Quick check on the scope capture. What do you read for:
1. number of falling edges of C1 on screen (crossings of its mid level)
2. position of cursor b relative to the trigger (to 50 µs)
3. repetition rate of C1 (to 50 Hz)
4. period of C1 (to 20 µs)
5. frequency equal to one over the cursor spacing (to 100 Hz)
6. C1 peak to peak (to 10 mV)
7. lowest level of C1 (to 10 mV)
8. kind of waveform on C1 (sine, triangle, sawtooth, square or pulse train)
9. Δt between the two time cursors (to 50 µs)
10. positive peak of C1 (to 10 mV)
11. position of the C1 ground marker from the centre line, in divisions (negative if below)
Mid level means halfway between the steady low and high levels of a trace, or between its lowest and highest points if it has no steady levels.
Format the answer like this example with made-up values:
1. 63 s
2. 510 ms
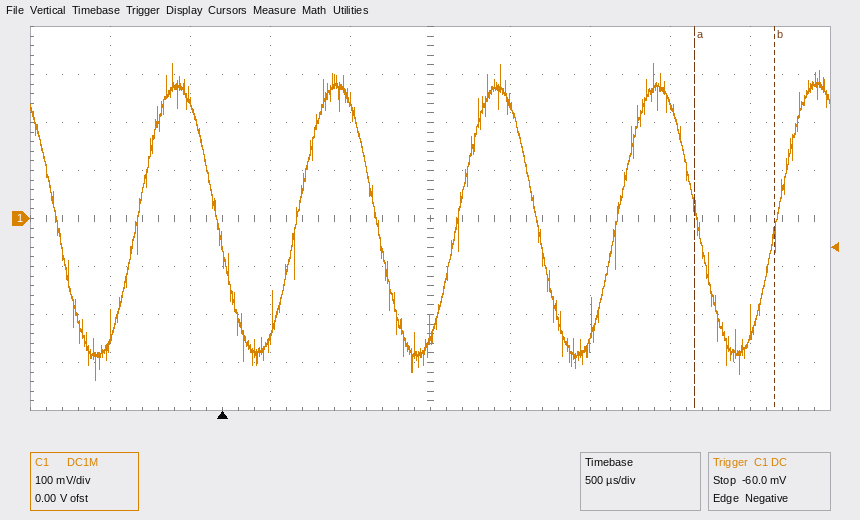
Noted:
1. 5
2. +3.45 ms
3. 1.00 kHz
4. 1.00 ms
5. 2.0 kHz
6. 660 mV
7. -340 mV
8. sine
9. 500 µs
10. 320 mV
11. 0.0 div
